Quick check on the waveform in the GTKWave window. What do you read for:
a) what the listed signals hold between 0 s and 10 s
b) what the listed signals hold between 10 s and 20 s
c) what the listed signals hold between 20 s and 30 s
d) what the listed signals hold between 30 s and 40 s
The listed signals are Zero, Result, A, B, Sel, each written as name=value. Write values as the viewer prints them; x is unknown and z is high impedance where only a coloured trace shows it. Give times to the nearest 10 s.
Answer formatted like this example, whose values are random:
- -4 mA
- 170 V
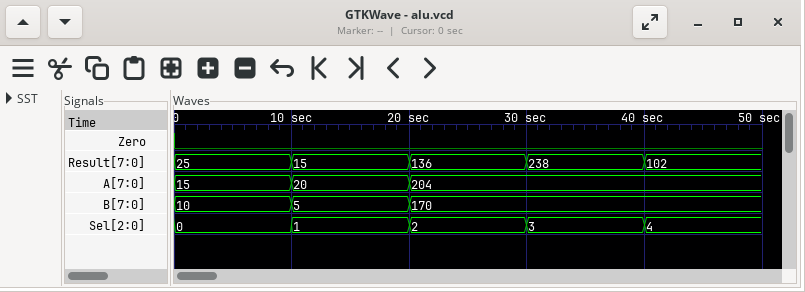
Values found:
- Zero=0, Result=25, A=15, B=10, Sel=0
- Zero=0, Result=15, A=20, B=5, Sel=1
- Zero=0, Result=136, A=204, B=170, Sel=2
- Zero=0, Result=238, A=204, B=170, Sel=3
